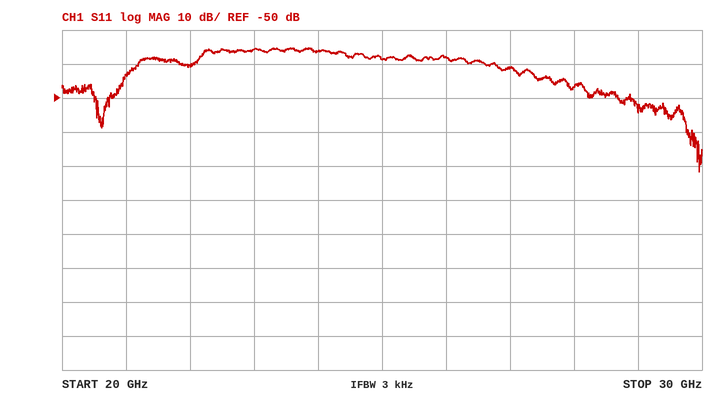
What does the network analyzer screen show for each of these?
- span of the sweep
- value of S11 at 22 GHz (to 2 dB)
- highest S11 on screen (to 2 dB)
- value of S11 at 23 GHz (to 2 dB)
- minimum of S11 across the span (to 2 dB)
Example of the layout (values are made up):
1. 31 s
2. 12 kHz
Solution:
1. 10 GHz
2. -40 dB
3. -36 dB
4. -36 dB
5. -72 dB
